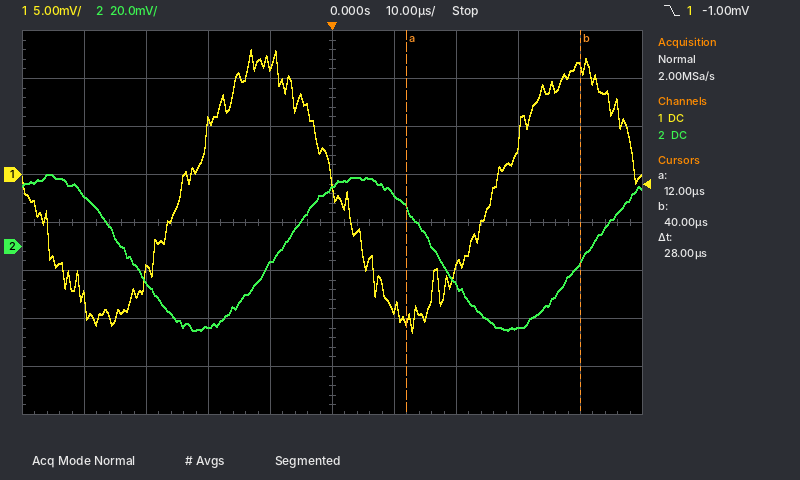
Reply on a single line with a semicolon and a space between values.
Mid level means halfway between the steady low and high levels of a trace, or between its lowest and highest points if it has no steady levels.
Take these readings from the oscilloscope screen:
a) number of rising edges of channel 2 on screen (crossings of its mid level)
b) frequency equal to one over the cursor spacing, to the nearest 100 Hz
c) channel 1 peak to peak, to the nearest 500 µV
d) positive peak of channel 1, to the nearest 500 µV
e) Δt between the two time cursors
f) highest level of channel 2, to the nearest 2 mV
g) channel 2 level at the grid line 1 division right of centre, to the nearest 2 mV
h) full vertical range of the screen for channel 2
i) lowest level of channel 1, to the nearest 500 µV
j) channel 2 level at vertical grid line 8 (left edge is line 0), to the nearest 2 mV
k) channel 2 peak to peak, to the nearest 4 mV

2; 35.7 kHz; 29.5 mV; 13.0 mV; 28 µs; 30 mV; 22 mV; 160 mV; -16.5 mV; -34 mV; 64 mV
